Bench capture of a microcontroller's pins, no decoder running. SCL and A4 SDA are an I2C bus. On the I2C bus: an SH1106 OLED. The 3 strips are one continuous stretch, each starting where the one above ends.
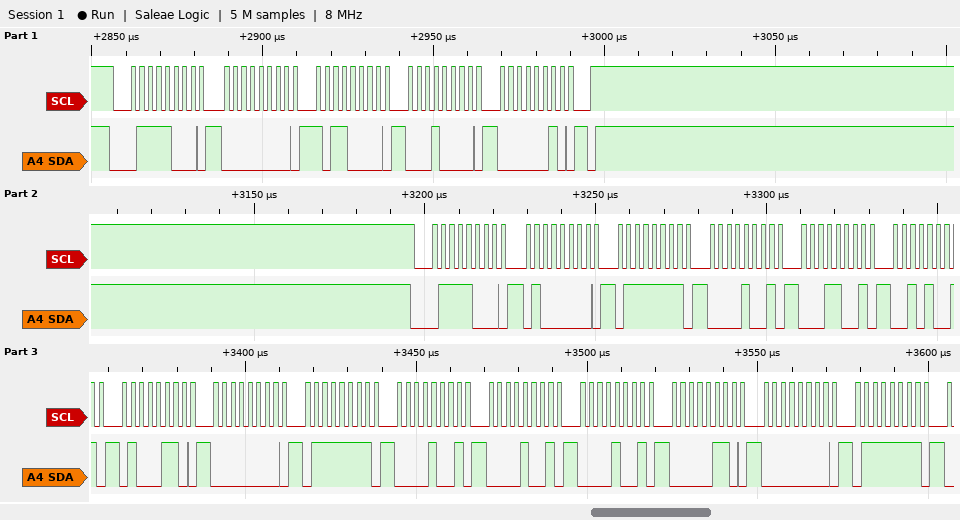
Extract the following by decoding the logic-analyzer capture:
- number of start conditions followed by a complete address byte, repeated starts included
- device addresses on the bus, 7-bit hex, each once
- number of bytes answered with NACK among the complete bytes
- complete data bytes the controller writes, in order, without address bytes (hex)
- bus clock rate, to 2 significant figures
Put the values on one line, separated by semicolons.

2; 0x3C; 0; 00 B0 10 02 40 7F 09 19 29 46 00 7F 09 09 09 06 00 7F; 400 kHz
